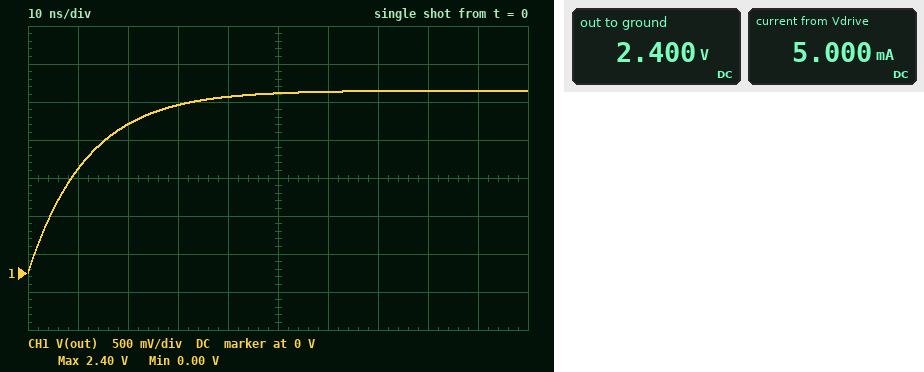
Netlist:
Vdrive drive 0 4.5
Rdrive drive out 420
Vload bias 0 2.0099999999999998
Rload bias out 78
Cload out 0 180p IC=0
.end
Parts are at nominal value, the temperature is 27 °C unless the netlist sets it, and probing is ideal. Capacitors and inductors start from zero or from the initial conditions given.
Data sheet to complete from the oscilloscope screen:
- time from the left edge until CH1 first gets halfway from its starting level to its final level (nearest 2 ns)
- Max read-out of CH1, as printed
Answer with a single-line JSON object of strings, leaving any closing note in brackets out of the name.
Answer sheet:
{"time from the left edge until CH1 first gets halfway from its starting level to its final level": "8 ns", "Max read-out of CH1, as printed": "2.40 V"}
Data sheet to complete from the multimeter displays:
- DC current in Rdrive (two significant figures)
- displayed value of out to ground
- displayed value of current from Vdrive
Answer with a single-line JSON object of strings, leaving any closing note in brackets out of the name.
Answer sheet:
{"DC current in Rdrive": "5.0 mA", "displayed value of out to ground": "2.400 V", "displayed value of current from Vdrive": "5.000 mA"}
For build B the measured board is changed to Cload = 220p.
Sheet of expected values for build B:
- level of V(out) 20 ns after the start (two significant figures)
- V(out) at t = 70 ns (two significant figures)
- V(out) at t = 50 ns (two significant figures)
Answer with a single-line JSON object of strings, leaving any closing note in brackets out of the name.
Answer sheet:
{"level of V(out) 20 ns after the start": "1.8 V", "V(out) at t = 70 ns": "2.4 V", "V(out) at t = 50 ns": "2.3 V"}
